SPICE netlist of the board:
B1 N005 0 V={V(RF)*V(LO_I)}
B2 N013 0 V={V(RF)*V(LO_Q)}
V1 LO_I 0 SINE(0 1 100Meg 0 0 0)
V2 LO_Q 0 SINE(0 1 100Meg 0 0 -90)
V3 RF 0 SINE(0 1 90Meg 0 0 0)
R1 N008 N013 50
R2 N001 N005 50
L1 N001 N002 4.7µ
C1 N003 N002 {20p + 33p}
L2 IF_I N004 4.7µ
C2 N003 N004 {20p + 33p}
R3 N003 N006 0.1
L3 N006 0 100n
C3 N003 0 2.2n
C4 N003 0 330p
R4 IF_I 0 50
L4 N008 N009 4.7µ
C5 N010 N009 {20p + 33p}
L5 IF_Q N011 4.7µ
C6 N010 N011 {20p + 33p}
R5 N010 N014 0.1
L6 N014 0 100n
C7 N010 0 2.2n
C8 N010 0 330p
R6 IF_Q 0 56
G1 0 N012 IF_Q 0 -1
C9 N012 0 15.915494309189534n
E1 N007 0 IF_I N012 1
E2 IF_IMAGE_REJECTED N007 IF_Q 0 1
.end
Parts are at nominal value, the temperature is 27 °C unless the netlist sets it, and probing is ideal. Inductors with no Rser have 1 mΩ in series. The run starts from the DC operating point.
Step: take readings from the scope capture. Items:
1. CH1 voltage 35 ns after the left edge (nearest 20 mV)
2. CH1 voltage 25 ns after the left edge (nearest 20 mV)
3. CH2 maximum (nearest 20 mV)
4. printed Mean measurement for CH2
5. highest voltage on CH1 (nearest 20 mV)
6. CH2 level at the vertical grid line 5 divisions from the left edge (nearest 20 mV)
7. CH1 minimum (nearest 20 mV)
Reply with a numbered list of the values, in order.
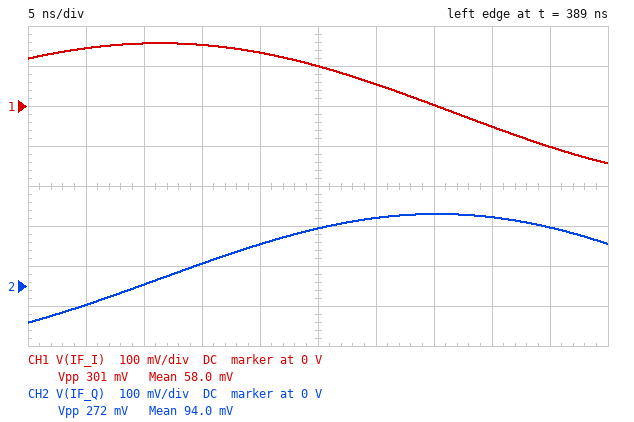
1. 0 V
2. 100 mV
3. 180 mV
4. 94.0 mV
5. 160 mV
6. 140 mV
7. -140 mV
